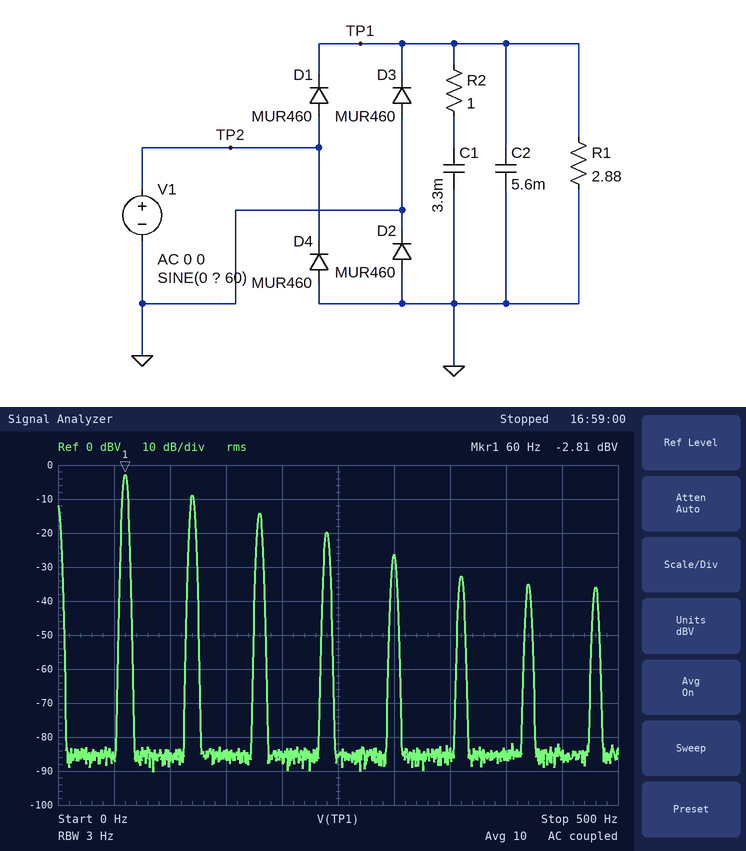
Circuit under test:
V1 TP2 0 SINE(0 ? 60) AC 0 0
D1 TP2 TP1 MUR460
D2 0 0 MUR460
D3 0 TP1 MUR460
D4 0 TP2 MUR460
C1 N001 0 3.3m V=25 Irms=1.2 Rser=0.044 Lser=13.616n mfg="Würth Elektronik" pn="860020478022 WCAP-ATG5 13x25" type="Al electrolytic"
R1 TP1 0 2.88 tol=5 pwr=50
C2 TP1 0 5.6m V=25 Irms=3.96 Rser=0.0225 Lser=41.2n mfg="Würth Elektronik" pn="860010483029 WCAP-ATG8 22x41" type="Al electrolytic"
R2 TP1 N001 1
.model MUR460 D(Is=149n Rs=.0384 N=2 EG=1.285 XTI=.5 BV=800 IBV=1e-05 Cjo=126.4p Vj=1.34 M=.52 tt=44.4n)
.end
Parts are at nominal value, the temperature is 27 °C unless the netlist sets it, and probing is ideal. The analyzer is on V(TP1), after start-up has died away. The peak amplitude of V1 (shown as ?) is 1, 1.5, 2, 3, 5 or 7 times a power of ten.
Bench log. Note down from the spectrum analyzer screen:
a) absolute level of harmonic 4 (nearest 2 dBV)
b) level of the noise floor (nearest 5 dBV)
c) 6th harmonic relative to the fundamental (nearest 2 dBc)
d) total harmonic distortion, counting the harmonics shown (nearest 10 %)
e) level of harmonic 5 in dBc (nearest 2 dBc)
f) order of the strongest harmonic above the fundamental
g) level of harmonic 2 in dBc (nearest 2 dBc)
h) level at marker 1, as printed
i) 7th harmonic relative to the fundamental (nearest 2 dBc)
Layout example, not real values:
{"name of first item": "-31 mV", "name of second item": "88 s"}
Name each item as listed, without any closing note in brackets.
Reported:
{"absolute level of harmonic 4": "-20 dBV", "level of the noise floor": "-85 dBV", "6th harmonic relative to the fundamental": "-30 dBc", "total harmonic distortion, counting the harmonics shown": "60 %", "level of harmonic 5 in dBc": "-24 dBc", "order of the strongest harmonic above the fundamental": "2", "level of harmonic 2 in dBc": "-6 dBc", "level at marker 1, as printed": "-2.81 dBV", "7th harmonic relative to the fundamental": "-32 dBc"}
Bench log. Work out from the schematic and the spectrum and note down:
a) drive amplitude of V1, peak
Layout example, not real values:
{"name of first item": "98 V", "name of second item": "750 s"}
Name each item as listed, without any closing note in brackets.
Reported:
{"drive amplitude of V1, peak": "7 V"}
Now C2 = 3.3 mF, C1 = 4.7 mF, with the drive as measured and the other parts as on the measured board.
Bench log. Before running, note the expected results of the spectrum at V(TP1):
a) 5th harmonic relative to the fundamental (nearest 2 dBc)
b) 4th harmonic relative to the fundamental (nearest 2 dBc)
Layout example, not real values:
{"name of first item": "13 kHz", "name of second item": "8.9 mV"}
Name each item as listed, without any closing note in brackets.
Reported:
{"5th harmonic relative to the fundamental": "-26 dBc", "4th harmonic relative to the fundamental": "-18 dBc"}
